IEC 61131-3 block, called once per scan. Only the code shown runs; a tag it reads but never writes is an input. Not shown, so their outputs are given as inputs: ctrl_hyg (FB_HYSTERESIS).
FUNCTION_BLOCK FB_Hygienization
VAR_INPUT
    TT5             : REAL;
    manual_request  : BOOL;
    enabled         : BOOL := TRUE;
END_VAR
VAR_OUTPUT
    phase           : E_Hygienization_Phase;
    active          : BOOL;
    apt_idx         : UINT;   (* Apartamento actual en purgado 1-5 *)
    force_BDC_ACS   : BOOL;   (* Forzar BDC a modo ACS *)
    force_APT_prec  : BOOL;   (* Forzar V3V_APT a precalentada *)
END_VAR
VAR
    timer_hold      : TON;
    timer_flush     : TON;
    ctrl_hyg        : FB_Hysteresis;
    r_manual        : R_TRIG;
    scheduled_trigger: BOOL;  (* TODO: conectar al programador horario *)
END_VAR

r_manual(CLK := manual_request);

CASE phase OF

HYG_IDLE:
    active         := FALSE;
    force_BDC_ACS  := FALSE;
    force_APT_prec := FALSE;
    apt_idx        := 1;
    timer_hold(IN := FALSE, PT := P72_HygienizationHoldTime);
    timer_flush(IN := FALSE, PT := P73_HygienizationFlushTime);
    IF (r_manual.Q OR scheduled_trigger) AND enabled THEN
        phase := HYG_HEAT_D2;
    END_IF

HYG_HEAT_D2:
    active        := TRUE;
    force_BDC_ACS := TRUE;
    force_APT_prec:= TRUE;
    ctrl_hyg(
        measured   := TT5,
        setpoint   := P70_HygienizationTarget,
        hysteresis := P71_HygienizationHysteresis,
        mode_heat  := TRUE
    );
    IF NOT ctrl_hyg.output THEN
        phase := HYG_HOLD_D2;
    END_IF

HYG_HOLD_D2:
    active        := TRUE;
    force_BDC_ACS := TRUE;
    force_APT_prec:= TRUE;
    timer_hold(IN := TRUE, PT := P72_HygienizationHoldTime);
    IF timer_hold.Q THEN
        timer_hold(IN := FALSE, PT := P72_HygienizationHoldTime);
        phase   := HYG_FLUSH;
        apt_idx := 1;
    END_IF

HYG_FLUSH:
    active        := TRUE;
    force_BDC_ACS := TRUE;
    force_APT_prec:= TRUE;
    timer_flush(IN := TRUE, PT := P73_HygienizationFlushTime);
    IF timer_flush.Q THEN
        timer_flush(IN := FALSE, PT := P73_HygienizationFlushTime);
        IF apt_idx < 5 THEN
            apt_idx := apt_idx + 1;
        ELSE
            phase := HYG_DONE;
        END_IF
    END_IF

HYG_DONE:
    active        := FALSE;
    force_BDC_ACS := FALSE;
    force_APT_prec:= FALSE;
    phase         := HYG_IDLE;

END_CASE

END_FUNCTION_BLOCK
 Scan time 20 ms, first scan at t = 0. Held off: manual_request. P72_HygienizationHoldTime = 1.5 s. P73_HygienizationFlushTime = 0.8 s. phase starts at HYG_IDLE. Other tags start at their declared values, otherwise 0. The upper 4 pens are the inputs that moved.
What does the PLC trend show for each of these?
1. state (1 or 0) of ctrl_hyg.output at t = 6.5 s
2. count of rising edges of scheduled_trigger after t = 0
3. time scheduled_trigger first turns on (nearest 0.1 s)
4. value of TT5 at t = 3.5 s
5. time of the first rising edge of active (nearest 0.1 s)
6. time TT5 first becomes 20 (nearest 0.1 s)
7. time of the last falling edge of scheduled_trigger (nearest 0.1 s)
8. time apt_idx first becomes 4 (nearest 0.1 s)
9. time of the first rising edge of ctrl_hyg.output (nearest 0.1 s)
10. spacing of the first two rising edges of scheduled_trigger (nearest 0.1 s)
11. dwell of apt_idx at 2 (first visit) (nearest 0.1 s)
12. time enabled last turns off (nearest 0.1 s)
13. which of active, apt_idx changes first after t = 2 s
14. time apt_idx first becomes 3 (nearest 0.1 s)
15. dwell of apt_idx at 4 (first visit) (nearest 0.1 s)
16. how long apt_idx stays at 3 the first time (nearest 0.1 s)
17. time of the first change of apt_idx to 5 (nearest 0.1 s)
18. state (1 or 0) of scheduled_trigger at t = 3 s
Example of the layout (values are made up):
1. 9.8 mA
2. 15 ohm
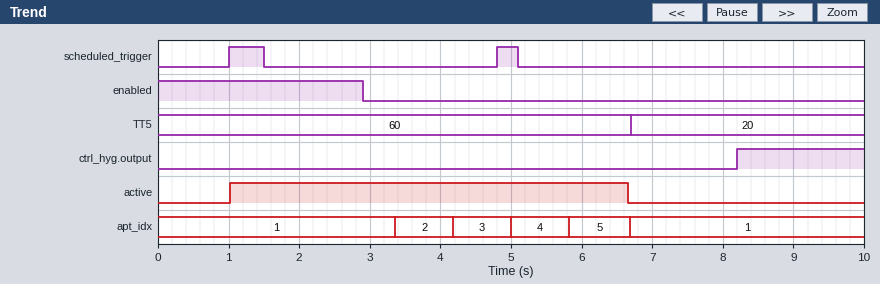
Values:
1. 0
2. 2
3. 1.0 s
4. 60
5. 1.0 s
6. 6.7 s
7. 5.1 s
8. 5.0 s
9. 8.2 s
10. 3.8 s
11. 0.8 s
12. 2.9 s
13. apt_idx
14. 4.2 s
15. 0.8 s
16. 0.8 s
17. 5.8 s
18. 0
